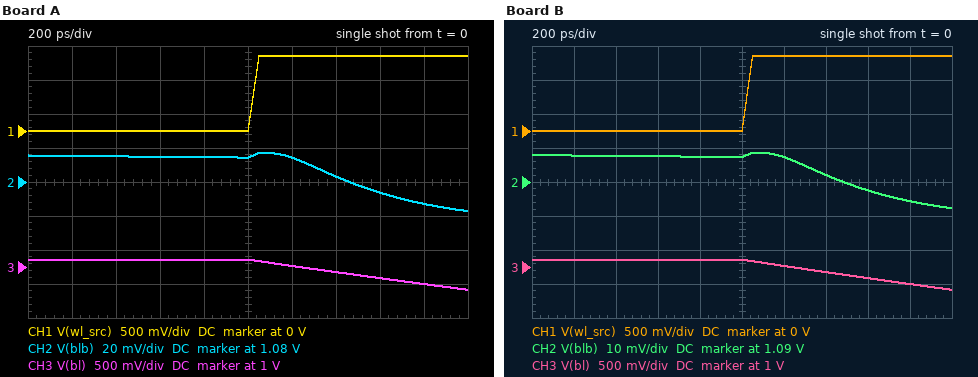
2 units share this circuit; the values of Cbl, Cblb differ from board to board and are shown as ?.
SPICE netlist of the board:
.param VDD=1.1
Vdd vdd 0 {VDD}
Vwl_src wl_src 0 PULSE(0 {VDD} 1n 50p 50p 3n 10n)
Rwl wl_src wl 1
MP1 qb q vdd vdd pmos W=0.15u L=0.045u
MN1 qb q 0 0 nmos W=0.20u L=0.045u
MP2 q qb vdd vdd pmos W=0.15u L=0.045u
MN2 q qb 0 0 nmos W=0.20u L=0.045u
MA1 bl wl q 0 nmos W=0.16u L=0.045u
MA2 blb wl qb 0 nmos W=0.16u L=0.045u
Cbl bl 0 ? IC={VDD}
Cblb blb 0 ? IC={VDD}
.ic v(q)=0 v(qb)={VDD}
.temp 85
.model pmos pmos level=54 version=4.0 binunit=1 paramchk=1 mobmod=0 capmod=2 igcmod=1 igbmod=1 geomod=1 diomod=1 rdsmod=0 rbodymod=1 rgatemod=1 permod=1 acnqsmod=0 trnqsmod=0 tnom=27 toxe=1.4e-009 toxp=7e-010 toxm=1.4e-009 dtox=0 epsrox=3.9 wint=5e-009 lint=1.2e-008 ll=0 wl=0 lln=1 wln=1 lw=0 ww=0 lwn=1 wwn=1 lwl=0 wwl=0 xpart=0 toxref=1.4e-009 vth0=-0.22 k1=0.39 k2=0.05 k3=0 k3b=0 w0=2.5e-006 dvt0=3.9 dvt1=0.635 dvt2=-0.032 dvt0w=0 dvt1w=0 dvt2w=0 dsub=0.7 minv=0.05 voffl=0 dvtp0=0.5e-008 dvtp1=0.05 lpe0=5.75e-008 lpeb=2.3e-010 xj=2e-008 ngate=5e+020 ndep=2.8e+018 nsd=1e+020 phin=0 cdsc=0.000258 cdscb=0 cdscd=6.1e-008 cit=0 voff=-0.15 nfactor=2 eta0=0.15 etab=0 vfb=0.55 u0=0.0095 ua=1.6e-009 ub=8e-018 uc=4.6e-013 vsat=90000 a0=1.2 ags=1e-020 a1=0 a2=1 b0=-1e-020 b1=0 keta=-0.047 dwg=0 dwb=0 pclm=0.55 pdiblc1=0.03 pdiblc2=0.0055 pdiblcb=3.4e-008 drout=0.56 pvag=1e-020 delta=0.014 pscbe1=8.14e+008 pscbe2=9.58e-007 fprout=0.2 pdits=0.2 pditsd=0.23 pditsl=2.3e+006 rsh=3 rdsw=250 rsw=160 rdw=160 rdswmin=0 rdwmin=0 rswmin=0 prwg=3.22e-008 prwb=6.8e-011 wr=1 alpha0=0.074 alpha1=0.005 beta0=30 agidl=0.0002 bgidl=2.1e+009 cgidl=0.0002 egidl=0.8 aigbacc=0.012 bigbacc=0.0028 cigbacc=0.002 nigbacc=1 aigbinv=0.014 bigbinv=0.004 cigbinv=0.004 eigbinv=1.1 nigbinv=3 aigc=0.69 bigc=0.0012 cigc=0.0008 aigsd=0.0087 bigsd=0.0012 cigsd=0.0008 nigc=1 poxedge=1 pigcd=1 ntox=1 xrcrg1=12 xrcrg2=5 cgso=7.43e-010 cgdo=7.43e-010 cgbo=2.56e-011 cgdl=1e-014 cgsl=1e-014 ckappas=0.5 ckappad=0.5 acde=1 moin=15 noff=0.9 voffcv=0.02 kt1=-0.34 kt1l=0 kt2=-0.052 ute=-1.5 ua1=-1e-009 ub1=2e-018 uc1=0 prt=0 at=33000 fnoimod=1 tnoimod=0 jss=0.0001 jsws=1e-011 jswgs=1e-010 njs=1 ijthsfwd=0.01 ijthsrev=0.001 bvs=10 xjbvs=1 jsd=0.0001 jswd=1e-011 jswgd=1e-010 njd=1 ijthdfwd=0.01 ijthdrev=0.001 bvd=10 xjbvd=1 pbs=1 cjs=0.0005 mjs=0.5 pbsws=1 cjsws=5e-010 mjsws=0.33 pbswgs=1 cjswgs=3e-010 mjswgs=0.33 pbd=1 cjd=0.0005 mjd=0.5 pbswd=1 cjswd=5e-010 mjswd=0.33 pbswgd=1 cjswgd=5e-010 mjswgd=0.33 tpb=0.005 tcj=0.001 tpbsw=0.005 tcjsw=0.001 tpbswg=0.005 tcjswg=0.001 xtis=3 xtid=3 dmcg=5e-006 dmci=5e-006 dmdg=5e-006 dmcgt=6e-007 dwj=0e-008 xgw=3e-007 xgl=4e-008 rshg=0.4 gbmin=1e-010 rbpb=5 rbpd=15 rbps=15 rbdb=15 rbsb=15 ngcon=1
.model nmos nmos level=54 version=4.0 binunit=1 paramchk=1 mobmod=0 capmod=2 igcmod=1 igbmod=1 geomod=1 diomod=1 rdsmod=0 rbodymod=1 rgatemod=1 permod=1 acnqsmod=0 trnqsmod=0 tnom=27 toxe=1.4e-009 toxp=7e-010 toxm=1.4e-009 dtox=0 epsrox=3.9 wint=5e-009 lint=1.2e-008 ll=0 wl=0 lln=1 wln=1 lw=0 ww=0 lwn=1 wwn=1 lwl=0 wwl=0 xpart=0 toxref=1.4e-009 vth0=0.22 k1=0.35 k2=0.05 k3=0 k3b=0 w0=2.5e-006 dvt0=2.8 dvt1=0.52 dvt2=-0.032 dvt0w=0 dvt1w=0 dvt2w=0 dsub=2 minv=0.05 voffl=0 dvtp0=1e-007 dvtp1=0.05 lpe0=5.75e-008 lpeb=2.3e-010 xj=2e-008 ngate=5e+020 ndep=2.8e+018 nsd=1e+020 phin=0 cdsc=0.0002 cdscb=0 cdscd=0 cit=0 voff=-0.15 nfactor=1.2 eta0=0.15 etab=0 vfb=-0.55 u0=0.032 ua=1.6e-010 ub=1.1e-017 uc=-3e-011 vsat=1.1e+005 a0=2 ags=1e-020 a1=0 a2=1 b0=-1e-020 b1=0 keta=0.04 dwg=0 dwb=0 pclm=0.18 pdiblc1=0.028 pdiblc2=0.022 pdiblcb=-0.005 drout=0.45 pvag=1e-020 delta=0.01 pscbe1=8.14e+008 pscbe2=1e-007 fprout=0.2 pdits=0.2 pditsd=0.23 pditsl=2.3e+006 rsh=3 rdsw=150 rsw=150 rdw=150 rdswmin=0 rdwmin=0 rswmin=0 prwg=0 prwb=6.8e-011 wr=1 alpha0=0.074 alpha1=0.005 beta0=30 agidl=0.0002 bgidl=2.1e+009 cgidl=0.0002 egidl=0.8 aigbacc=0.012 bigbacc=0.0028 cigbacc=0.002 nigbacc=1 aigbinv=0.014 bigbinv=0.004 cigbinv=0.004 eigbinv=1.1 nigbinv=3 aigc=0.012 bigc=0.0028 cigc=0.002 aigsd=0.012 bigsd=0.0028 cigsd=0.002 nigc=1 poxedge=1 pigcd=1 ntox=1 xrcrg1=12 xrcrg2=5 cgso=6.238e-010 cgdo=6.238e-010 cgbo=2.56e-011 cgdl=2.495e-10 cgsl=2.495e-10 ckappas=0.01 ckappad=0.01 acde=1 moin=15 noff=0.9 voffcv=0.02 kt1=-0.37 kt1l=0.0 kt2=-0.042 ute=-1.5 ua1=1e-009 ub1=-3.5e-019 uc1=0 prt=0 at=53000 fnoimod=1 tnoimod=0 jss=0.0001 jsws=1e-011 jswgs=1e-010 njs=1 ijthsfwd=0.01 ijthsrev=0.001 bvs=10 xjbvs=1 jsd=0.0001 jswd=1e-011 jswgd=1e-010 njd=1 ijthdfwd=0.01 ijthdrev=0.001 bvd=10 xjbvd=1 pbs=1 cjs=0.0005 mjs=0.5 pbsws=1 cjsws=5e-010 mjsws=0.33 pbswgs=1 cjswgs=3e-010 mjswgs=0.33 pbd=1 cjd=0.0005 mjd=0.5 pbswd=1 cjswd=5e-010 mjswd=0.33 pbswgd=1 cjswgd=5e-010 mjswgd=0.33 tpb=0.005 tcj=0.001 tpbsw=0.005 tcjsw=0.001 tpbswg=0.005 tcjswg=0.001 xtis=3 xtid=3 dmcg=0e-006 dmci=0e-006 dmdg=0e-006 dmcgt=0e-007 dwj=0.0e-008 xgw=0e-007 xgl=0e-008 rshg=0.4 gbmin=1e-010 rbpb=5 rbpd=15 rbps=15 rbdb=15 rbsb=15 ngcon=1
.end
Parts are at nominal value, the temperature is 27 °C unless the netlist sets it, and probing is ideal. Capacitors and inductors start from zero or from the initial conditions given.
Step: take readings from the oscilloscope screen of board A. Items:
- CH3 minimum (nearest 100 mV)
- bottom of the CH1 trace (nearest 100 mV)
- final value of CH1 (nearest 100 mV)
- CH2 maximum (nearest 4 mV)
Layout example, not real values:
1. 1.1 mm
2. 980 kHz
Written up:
1. 700 mV
2. 0 V
3. 1.1 V
4. 1.096 V
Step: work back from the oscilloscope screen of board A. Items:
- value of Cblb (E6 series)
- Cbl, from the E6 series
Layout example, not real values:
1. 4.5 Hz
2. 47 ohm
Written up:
1. 47 fF
2. 220 fF
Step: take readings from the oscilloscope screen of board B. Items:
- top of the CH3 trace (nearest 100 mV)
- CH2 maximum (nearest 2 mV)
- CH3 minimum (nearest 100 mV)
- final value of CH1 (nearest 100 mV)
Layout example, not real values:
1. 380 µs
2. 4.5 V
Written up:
1. 1.1 V
2. 1.098 V
3. 700 mV
4. 1.1 V
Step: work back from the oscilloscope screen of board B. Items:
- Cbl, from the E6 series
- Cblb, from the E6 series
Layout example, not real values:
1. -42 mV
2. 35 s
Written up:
1. 220 fF
2. 100 fF
